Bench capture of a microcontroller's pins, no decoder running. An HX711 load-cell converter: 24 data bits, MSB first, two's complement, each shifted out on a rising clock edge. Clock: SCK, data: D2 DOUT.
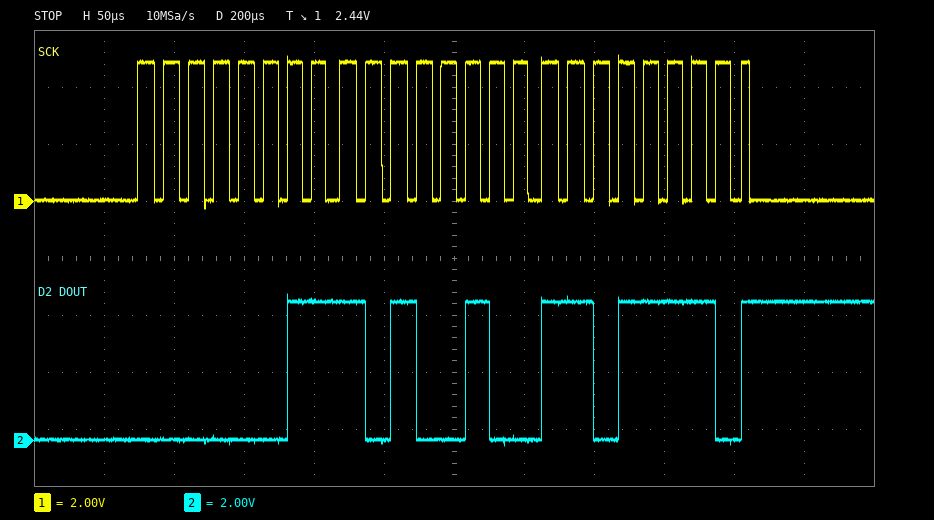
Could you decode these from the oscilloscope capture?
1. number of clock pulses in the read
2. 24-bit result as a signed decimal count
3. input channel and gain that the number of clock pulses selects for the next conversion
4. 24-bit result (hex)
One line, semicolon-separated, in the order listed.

25; 238814; channel A, gain 128; 0x03A4DE
